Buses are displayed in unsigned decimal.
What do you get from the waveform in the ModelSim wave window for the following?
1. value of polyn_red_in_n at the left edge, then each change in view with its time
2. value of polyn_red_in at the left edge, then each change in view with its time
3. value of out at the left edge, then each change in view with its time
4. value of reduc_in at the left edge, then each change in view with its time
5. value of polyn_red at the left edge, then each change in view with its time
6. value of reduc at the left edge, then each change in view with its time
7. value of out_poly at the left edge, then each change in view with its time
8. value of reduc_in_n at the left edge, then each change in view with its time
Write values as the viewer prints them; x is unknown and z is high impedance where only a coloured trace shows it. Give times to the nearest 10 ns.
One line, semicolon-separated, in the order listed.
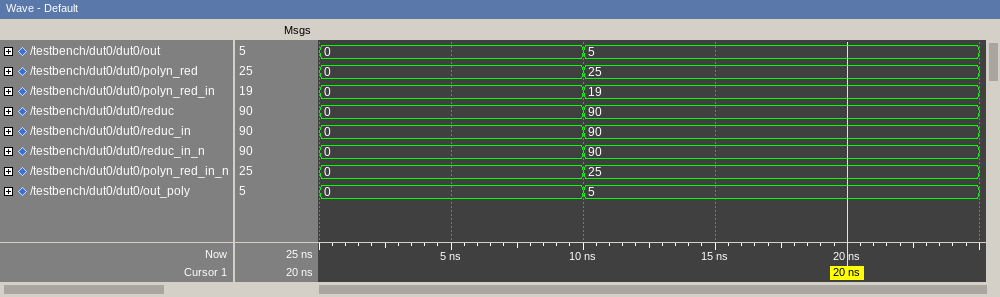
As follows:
0, 25 at 10 ns; 0, 19 at 10 ns; 0, 5 at 10 ns; 0, 90 at 10 ns; 0, 25 at 10 ns; 0, 90 at 10 ns; 0, 5 at 10 ns; 0, 90 at 10 ns
